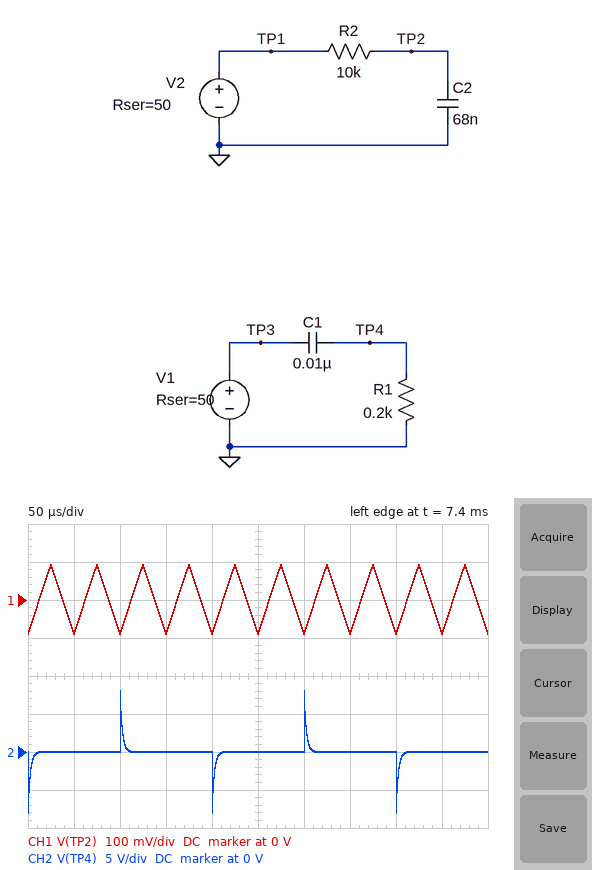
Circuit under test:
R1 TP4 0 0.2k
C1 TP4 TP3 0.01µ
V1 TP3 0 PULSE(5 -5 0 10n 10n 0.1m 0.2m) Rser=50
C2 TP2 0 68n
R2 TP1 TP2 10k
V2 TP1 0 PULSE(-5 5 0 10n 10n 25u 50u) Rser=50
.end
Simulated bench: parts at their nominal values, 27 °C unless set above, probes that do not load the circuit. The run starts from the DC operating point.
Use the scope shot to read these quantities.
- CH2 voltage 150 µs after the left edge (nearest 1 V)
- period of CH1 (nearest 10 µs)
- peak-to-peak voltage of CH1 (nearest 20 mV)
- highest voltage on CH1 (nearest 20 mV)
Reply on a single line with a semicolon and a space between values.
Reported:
0 V; 50 µs; 180 mV; 100 mV
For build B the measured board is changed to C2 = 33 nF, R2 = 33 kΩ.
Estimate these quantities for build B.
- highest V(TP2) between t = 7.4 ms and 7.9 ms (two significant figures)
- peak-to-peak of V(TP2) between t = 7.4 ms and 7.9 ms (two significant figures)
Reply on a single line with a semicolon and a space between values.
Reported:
56 mV; 120 mV
